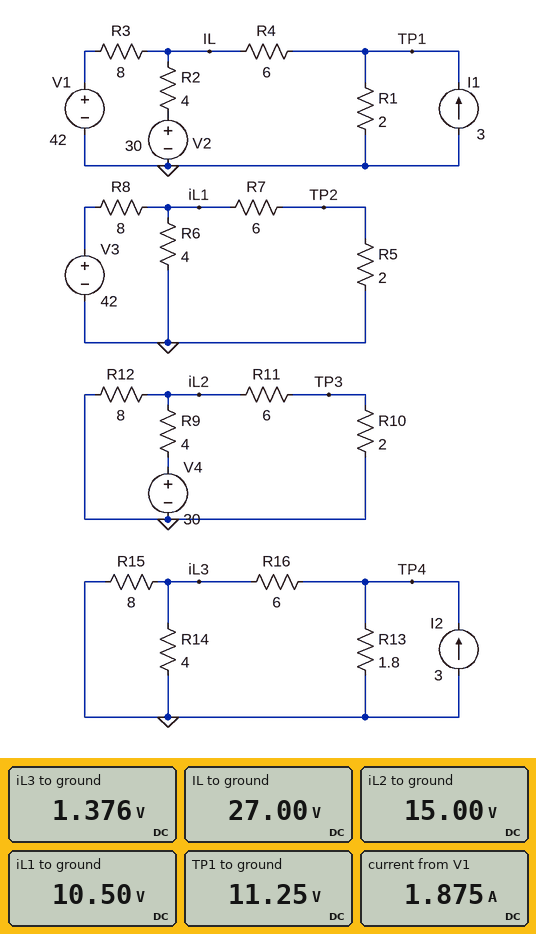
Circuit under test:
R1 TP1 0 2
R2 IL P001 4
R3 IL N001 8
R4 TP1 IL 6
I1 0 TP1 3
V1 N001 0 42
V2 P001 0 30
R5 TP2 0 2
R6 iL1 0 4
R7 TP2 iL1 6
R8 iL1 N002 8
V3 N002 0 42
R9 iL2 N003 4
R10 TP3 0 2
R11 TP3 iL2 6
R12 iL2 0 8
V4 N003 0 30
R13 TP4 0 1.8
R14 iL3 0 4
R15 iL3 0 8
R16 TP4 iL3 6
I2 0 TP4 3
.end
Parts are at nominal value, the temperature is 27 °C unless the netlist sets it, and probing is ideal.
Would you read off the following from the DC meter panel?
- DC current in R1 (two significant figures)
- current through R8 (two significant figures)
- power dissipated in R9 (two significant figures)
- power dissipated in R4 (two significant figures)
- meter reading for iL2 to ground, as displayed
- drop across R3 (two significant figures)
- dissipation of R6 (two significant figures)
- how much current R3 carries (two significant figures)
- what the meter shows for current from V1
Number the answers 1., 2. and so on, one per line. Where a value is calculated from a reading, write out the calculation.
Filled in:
1. (11.25 V) / 2 Ω = 5.6 A
2. (42 V - 10.5 V) / 8 Ω = 3.9 A
3. (30 V - 15 V)^2 / 4 Ω = 56 W
4. (27 V - 11.25 V)^2 / 6 Ω = 41 W
5. 15.00 V
6. 42 V - 27 V = 15 V
7. (10.5 V)^2 / 4 Ω = 28 W
8. (42 V - 27 V) / 8 Ω = 1.9 A
9. 1.875 A
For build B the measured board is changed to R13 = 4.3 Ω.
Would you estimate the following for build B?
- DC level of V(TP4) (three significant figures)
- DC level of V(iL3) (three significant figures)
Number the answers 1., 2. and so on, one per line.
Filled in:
1. 8.62 V
2. 2.65 V
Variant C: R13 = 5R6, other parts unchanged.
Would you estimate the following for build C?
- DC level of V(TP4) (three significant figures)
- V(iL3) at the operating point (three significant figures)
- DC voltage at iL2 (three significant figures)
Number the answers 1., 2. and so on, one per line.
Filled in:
1. 10.2 V
2. 3.14 V
3. 15.0 V
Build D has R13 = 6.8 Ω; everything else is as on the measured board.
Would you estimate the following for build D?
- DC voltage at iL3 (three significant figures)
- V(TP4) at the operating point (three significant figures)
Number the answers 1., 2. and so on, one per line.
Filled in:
1. 3.52 V
2. 11.4 V
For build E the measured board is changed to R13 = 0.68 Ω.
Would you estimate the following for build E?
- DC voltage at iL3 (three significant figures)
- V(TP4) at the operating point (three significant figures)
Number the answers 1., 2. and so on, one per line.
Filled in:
1. 582 mV
2. 1.89 V
